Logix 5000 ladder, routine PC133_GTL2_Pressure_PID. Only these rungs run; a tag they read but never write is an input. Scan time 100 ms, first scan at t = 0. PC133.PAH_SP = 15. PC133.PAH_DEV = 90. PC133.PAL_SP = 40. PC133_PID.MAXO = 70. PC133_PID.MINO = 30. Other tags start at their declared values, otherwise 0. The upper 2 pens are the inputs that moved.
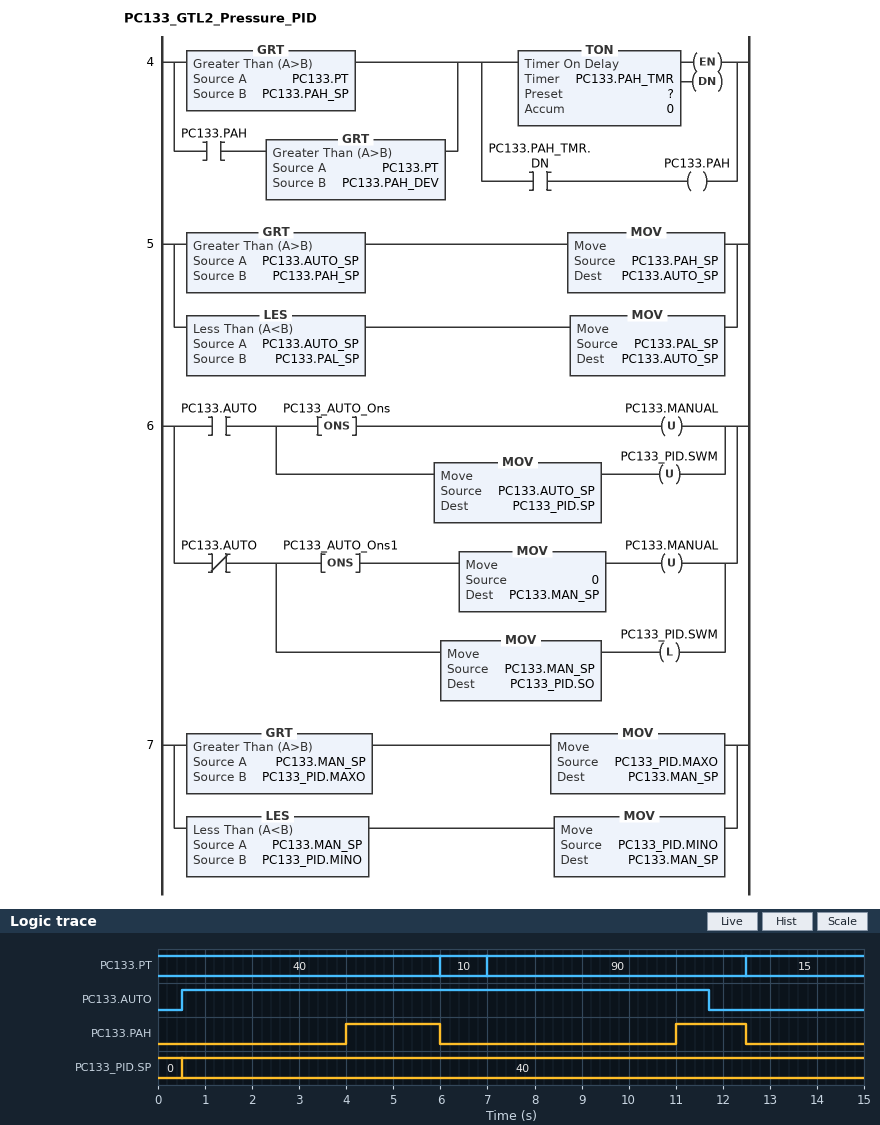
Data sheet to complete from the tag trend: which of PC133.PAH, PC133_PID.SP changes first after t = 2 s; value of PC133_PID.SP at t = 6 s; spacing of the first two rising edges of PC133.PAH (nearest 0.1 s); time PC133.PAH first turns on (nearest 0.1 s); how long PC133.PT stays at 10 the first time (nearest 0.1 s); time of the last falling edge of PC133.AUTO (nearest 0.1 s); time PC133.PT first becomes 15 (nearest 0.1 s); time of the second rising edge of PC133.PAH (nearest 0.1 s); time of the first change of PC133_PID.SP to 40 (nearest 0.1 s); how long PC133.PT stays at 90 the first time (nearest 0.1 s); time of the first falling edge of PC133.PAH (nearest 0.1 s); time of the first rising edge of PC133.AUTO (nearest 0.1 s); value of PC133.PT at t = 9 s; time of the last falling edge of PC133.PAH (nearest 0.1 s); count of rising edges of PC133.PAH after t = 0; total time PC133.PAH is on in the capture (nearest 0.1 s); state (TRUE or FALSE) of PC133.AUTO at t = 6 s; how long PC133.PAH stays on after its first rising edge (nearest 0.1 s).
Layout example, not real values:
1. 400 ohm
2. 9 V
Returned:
1. PC133.PAH
2. 40
3. 7.0 s
4. 4.0 s
5. 1.0 s
6. 11.7 s
7. 12.5 s
8. 11.0 s
9. 0.5 s
10. 5.5 s
11. 6.0 s
12. 0.5 s
13. 90
14. 12.5 s
15. 2
16. 3.5 s
17. TRUE
18. 2.0 s
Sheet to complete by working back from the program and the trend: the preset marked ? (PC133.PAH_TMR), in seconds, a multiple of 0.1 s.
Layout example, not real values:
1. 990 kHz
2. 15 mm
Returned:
1. 4.0 s
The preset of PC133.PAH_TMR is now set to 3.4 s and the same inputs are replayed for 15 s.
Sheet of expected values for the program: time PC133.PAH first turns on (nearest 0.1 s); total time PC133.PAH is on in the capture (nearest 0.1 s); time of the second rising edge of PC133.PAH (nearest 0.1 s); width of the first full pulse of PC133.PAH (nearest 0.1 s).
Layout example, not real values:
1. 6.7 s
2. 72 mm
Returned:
1. 3.4 s
2. 4.7 s
3. 10.4 s
4. 2.6 s
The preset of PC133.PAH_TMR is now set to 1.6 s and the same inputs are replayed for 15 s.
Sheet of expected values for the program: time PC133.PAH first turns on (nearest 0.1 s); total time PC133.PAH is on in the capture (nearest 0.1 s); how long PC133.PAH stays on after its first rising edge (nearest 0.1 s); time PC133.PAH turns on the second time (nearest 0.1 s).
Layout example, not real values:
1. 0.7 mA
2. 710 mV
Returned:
1. 1.6 s
2. 8.3 s
3. 4.4 s
4. 8.6 s
